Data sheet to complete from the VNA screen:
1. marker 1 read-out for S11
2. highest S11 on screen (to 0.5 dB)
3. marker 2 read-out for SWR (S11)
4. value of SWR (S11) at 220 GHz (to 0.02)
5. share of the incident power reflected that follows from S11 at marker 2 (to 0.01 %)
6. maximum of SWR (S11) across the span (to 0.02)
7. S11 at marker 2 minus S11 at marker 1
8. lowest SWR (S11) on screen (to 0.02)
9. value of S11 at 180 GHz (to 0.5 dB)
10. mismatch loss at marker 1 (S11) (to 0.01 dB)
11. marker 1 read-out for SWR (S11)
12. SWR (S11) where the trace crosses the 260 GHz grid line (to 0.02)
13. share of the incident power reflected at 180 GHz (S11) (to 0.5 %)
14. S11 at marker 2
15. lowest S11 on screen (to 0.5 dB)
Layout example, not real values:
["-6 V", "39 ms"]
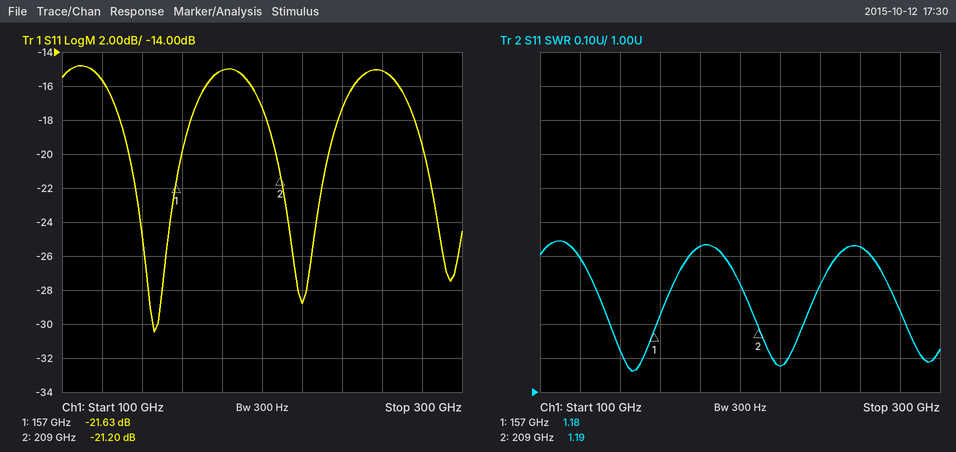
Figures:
["-21.63 dB", "-15.0 dB", "1.19", "1.08", "0.76 %", "1.44", "0.43 dB", "1.06", "-15.0 dB", "0.03 dB", "1.18", "1.42", "3.0 %", "-21.20 dB", "-30.5 dB"]
